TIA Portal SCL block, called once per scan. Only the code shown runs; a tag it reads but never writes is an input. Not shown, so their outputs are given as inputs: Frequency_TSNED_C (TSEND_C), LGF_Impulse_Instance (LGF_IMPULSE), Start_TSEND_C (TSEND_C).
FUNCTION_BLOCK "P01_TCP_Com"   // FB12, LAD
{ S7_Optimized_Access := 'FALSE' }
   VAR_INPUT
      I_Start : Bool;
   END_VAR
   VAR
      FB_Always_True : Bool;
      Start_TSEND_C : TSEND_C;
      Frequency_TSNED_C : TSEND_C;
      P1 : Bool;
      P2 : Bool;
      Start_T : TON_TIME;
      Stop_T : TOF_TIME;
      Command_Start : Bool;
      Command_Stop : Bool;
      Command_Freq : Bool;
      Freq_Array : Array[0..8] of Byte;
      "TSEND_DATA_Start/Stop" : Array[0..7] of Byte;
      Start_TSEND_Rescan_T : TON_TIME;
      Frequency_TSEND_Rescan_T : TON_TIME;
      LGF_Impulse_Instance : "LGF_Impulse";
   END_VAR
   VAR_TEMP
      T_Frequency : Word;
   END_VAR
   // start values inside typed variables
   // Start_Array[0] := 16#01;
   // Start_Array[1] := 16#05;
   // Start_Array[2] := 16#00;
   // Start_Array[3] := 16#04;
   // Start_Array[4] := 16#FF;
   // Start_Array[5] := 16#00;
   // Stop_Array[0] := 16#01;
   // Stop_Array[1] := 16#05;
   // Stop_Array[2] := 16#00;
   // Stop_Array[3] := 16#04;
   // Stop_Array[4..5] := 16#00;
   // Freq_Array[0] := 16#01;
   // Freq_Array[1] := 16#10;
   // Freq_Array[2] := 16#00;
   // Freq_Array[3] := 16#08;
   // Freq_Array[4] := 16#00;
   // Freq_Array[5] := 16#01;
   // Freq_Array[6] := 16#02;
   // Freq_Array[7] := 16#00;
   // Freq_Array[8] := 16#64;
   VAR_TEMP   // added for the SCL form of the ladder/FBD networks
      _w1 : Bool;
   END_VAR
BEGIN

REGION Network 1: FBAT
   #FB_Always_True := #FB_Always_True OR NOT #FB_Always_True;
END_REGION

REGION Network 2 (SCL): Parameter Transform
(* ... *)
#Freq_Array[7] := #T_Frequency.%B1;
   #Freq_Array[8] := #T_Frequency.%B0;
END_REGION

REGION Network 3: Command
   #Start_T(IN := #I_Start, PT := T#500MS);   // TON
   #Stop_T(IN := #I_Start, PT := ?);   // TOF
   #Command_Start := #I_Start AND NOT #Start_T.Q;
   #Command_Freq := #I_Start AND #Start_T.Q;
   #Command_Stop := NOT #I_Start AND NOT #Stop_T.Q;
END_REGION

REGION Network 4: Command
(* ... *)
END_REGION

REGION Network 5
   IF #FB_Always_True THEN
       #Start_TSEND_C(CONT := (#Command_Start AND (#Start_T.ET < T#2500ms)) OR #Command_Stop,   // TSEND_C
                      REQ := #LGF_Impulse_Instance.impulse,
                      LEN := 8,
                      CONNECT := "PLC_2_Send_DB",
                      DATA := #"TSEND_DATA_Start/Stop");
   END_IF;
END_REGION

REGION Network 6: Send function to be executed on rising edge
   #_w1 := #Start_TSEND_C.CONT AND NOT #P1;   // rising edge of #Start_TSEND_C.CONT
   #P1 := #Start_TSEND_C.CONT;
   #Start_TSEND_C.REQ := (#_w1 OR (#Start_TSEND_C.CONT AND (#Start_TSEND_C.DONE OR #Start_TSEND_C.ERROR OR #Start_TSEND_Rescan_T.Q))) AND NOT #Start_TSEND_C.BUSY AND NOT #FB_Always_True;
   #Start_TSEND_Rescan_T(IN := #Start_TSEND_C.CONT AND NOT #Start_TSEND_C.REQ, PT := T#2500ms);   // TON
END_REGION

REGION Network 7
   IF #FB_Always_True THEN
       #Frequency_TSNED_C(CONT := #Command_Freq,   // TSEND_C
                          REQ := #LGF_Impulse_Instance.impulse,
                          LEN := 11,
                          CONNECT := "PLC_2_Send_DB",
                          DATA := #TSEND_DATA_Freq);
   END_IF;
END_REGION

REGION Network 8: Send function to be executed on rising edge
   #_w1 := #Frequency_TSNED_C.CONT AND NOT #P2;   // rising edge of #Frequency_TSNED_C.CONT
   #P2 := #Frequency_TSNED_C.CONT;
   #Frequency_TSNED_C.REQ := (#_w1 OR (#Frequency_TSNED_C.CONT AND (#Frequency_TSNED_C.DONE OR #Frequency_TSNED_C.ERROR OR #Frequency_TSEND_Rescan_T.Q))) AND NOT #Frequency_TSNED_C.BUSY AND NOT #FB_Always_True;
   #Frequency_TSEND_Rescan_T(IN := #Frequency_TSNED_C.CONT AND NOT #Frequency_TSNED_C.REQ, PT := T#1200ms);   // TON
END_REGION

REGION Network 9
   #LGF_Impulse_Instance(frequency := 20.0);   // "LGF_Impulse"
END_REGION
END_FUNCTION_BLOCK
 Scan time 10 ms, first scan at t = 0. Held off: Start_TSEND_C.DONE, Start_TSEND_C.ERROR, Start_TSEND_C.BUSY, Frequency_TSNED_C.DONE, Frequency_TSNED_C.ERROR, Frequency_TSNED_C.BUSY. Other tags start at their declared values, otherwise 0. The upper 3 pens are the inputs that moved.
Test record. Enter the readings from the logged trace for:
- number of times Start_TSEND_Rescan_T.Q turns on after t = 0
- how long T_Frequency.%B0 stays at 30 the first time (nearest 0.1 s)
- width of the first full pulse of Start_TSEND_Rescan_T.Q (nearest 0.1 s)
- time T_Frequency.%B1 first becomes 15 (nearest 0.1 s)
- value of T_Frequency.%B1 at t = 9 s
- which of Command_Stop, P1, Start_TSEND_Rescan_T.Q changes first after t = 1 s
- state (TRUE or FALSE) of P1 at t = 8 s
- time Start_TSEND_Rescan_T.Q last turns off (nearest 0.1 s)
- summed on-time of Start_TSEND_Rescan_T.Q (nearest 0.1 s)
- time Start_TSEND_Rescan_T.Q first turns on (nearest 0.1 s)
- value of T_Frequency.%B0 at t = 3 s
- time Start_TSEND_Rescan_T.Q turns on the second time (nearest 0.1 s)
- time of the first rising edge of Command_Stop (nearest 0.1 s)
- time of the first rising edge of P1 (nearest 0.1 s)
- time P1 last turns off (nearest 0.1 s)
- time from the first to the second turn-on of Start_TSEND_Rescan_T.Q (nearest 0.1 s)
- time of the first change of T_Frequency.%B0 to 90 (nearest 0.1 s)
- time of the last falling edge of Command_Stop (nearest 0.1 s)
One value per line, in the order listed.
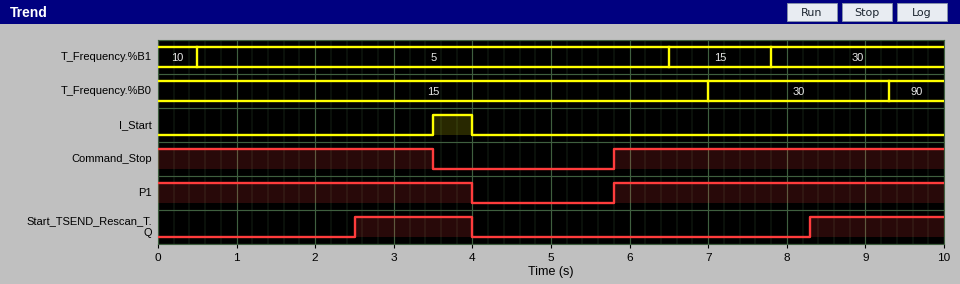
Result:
2
2.3 s
1.5 s
6.5 s
30
Start_TSEND_Rescan_T.Q
TRUE
4.0 s
3.2 s
2.5 s
15
8.3 s
5.8 s
5.8 s
4.0 s
5.8 s
9.3 s
3.5 s
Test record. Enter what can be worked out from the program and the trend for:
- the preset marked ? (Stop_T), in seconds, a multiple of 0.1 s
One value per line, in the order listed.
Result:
1.8 s
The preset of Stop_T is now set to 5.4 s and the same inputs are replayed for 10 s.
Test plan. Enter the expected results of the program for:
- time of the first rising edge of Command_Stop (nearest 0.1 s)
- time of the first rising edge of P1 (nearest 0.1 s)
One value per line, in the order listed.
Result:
9.4 s
9.4 s
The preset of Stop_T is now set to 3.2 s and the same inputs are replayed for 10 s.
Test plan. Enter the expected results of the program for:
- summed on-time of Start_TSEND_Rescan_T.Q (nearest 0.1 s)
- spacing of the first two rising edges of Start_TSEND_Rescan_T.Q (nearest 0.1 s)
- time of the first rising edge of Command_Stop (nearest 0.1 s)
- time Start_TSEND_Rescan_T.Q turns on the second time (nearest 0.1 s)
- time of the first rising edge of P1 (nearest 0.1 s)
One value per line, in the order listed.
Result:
1.8 s
7.2 s
7.2 s
9.7 s
7.2 s
